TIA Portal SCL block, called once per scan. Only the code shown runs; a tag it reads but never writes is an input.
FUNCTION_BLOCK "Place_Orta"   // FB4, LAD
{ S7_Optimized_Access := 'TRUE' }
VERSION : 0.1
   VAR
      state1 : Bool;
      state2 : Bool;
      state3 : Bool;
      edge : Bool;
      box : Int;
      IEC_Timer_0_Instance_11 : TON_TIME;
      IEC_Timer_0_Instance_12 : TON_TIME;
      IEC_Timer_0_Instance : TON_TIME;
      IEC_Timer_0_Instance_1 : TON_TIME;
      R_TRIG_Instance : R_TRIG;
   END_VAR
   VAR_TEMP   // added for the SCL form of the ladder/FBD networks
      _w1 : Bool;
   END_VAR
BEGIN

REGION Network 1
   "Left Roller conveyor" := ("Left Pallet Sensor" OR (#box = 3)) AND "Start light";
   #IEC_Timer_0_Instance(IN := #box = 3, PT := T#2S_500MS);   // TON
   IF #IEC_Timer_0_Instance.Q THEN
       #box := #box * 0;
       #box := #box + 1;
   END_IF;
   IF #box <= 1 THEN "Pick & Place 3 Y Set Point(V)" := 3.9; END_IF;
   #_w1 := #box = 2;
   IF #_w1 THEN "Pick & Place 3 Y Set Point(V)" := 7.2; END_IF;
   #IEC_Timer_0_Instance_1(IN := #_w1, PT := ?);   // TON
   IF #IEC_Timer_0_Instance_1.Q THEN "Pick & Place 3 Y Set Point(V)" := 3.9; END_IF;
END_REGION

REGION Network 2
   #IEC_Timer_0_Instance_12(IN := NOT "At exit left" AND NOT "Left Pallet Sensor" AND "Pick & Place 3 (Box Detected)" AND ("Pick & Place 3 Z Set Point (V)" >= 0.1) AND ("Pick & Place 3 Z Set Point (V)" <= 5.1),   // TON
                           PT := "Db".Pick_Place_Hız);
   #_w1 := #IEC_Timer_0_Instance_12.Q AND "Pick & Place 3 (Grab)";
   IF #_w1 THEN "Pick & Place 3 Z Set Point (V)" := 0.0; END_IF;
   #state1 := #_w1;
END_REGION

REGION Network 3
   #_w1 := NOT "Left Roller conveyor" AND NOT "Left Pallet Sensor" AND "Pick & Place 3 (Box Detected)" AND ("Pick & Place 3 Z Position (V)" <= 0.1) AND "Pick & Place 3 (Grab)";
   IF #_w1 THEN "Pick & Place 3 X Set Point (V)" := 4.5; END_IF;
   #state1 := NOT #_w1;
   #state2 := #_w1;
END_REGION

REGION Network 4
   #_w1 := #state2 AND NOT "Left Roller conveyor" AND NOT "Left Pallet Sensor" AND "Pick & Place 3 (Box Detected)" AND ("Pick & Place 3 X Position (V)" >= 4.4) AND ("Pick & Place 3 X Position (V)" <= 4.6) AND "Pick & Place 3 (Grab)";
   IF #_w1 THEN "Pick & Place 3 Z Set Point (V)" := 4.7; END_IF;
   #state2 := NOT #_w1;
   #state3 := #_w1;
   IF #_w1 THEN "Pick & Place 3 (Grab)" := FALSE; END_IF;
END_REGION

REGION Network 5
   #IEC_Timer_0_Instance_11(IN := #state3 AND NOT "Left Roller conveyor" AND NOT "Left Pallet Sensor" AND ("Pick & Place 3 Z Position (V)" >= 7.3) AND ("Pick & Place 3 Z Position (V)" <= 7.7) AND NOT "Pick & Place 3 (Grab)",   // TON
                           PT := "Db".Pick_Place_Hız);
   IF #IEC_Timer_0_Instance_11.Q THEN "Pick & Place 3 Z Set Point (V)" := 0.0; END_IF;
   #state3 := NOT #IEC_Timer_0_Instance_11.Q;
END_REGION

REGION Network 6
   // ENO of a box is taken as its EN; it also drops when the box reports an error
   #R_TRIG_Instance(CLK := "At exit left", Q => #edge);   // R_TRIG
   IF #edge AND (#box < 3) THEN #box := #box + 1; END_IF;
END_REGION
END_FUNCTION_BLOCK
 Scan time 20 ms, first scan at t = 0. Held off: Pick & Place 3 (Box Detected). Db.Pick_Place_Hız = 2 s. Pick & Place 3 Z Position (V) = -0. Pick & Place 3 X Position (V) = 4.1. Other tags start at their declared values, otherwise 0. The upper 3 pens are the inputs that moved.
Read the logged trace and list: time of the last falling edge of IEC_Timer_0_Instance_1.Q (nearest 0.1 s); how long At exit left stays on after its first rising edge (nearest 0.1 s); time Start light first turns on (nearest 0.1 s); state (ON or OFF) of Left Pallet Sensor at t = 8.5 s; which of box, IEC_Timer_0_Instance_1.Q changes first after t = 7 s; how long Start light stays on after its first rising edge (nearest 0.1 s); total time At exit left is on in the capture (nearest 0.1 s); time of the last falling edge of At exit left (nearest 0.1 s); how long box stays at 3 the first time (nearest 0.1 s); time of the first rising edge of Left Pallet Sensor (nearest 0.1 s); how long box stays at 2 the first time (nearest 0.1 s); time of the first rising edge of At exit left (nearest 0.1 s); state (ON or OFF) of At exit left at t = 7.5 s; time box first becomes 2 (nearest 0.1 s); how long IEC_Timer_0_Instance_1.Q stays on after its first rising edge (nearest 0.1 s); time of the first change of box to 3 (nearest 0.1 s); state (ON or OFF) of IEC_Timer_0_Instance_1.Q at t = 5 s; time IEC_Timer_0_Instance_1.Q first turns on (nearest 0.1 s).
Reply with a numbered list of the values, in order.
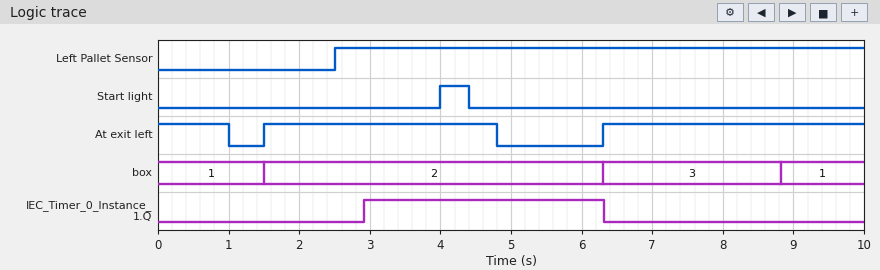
1. 6.3 s
2. 3.3 s
3. 4.0 s
4. ON
5. box
6. 0.4 s
7. 8.0 s
8. 4.8 s
9. 2.5 s
10. 2.5 s
11. 4.8 s
12. 1.5 s
13. ON
14. 1.5 s
15. 3.4 s
16. 6.3 s
17. ON
18. 2.9 s
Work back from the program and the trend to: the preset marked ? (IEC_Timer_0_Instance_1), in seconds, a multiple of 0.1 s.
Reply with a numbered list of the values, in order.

1. 1.4 s
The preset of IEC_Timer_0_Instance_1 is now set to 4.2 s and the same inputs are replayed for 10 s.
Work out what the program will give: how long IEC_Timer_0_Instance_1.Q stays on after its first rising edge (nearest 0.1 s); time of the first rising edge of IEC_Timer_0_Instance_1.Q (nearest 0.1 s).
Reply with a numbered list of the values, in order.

1. 0.6 s
2. 5.7 s
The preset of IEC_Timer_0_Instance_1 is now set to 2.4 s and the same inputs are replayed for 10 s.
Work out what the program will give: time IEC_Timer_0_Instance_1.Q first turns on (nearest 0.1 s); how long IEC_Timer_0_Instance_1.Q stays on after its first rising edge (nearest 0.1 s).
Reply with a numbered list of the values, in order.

1. 3.9 s
2. 2.4 s
